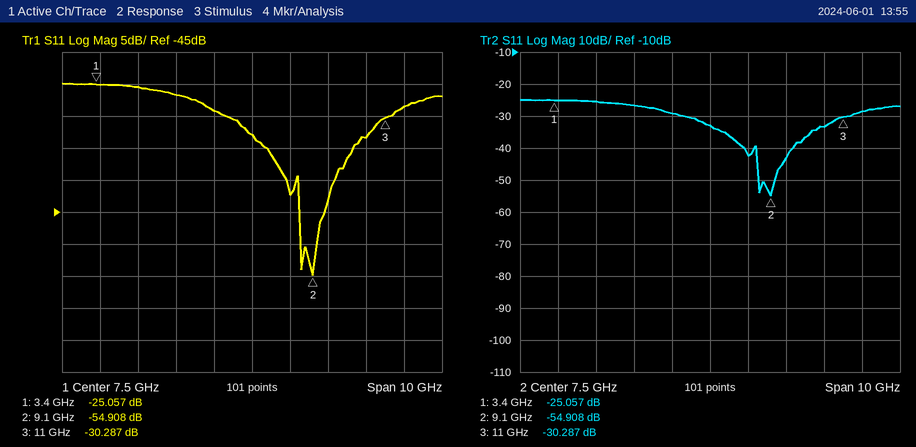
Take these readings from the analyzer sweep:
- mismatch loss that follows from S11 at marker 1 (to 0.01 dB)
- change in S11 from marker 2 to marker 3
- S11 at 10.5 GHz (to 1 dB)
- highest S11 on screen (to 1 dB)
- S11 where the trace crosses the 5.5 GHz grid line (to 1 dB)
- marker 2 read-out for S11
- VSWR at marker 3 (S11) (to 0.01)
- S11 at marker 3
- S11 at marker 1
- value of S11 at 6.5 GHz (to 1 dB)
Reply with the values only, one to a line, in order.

0.01 dB
24.621 dB
-33 dB
-25 dB
-27 dB
-54.908 dB
1.06
-30.287 dB
-25.057 dB
-29 dB
